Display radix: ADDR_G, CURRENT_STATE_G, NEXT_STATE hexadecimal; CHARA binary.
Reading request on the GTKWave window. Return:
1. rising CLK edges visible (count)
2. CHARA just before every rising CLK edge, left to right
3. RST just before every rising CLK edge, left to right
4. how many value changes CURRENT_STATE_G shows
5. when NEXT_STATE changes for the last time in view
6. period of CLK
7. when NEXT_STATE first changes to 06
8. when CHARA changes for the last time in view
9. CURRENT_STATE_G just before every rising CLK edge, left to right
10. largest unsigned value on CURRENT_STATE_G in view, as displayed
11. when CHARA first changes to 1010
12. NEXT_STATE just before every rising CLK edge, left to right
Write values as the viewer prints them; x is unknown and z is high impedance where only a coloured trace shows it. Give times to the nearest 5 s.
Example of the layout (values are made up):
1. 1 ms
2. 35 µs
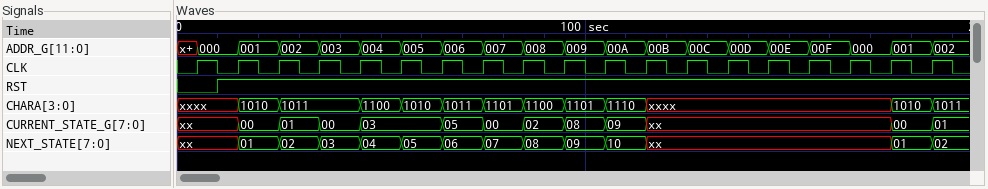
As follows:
1. 19
2. xxxx, xxxx, 1010, 1011, 1011, 1100, 1010, 1011, 1101, 1100, 1101, 1110, xxxx, xxxx, xxxx, xxxx, xxxx, xxxx, 1010
3. 0 1 1 1 1 1 1 1 1 1 1 1 1 1 1 1 1 1 1
4. 12
5. 185 s
6. 10 s
7. 65 s
8. 185 s
9. xx, xx, 00, 01, 00, 03, 03, 05, 00, 02, 08, 09, xx, xx, xx, xx, xx, xx, 00
10. 09
11. 15 s
12. xx, xx, 01, 02, 03, 04, 05, 06, 07, 08, 09, 10, xx, xx, xx, xx, xx, xx, 01
